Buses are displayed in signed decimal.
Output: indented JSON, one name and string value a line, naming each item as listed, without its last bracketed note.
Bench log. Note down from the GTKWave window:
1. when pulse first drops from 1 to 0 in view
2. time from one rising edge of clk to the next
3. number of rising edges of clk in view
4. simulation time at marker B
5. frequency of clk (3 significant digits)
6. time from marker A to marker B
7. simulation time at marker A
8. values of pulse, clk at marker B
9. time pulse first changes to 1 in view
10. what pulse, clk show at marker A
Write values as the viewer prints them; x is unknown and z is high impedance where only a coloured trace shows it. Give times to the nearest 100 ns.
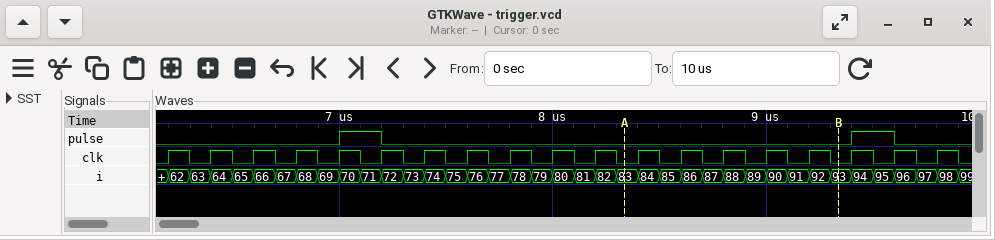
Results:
{
  "when pulse first drops from 1 to 0 in view": "7200 ns",
  "time from one rising edge of clk to the next": "200 ns",
  "number of rising edges of clk in view": "19",
  "simulation time at marker B": "9300 ns",
  "frequency of clk": "5.00 MHz",
  "time from marker A to marker B": "1000 ns",
  "simulation time at marker A": "8300 ns",
  "values of pulse, clk at marker B": "pulse=0, clk=0",
  "time pulse first changes to 1 in view": "7000 ns",
  "what pulse, clk show at marker A": "pulse=0, clk=0"
}
